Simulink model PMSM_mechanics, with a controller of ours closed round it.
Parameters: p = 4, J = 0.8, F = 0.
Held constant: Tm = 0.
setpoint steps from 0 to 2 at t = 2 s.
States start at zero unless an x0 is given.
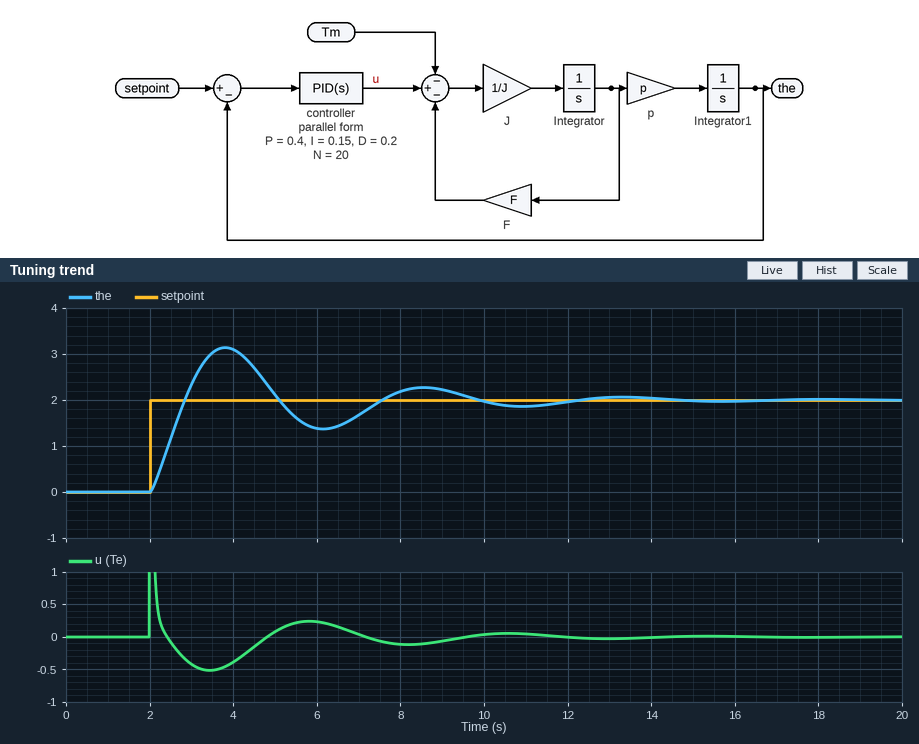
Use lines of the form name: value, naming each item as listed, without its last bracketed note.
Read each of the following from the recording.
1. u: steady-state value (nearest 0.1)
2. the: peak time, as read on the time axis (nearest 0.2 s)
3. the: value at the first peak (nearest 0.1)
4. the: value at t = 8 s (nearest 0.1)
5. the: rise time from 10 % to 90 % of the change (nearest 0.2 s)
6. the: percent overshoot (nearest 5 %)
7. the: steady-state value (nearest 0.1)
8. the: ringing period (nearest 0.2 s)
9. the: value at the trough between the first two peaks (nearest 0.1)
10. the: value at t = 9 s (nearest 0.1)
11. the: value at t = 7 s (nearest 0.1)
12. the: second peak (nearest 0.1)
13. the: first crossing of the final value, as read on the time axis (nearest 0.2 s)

u: steady-state value: 0.0
the: peak time, as read on the time axis: 3.8 s
the: value at the first peak: 3.1
the: value at t = 8 s: 2.2
the: rise time from 10 % to 90 % of the change: 0.6 s
the: percent overshoot: 55 %
the: steady-state value: 2.0
the: ringing period: 4.8 s
the: value at the trough between the first two peaks: 1.4
the: value at t = 9 s: 2.2
the: value at t = 7 s: 1.7
the: second peak: 2.3
the: first crossing of the final value, as read on the time axis: 2.8 s
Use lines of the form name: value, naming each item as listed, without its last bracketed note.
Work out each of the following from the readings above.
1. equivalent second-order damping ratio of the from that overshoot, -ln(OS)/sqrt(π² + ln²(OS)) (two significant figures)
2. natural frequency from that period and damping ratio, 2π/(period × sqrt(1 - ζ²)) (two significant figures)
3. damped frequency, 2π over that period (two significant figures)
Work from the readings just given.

equivalent second-order damping ratio of the from that overshoot, -ln(OS)/sqrt(π² + ln²(OS)): 0.19
natural frequency from that period and damping ratio, 2π/(period × sqrt(1 - ζ²)): 1.3 rad/s
damped frequency, 2π over that period: 1.3 rad/s
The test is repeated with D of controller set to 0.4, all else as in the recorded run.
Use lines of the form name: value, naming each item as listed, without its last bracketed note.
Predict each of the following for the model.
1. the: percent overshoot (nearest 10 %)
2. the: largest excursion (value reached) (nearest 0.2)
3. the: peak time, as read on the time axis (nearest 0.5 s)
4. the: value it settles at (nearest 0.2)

the: percent overshoot: 30 %
the: largest excursion (value reached): 2.6
the: peak time, as read on the time axis: 3.5 s
the: value it settles at: 2.0
